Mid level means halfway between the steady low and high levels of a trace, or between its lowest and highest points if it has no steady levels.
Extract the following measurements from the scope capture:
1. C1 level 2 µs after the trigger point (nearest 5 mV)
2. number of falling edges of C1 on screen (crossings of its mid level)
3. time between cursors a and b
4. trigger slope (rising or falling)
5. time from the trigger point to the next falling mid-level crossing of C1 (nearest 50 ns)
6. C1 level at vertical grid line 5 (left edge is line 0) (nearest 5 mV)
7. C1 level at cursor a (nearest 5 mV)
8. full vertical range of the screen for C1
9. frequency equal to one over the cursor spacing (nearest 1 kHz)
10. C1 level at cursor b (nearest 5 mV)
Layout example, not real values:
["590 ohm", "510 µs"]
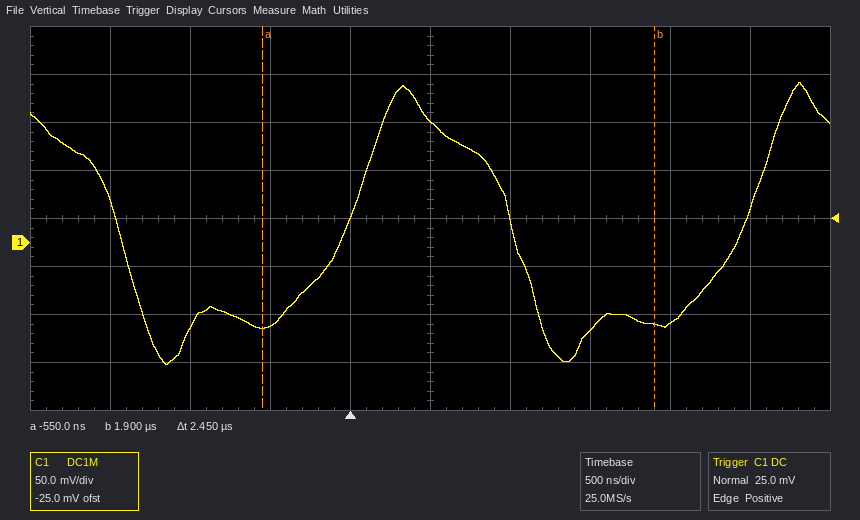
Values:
["-85 mV", "2", "2.45 µs", "rising", "1.00 µs", "125 mV", "-90 mV", "400 mV", "408 kHz", "-85 mV"]
